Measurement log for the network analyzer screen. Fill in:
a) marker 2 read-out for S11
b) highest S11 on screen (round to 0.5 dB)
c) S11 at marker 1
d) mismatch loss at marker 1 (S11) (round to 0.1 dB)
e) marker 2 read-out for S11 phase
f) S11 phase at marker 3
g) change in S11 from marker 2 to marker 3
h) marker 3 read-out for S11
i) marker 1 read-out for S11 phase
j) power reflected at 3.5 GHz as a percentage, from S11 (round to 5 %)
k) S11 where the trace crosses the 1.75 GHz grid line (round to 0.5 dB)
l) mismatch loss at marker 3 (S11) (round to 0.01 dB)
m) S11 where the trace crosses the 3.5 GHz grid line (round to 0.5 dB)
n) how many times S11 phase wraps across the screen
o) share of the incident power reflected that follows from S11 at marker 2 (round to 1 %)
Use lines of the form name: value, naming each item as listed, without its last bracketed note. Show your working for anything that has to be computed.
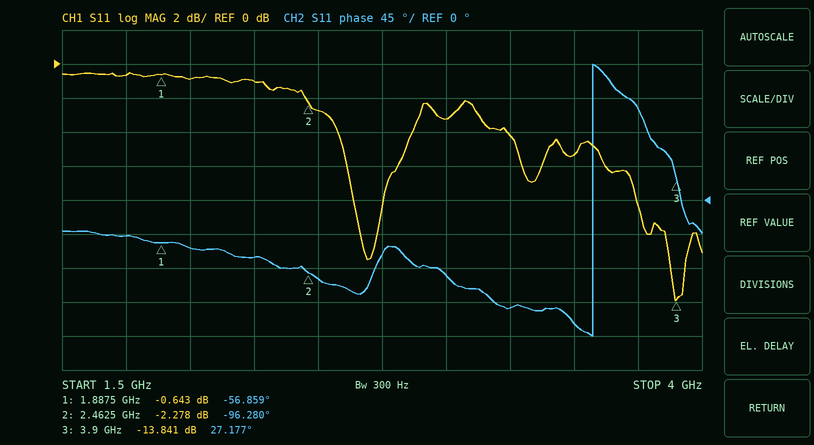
marker 2 read-out for S11: -2.278 dB
highest S11 on screen: -0.5 dB
S11 at marker 1: -0.643 dB
mismatch loss at marker 1 (S11): −10 log10(1 − 10^(-0.643/10)) ≈ 8.6 dB
marker 2 read-out for S11 phase: -96.280°
S11 phase at marker 3: 27.177°
change in S11 from marker 2 to marker 3: -13.841 − (-2.278) = -11.563 dB
marker 3 read-out for S11: -13.841 dB
marker 1 read-out for S11 phase: -56.859°
power reflected at 3.5 GHz as a percentage, from S11: 10^(-5.5/10) ≈ 28.2 %, so 30 % to the nearest 5 %
S11 where the trace crosses the 1.75 GHz grid line: -0.5 dB
mismatch loss at marker 3 (S11): −10 log10(1 − 10^(-13.841/10)) ≈ 0.18 dB
S11 where the trace crosses the 3.5 GHz grid line: -5.5 dB
how many times S11 phase wraps across the screen: 1
share of the incident power reflected that follows from S11 at marker 2: 10^(-2.278/10) ≈ 59 %
